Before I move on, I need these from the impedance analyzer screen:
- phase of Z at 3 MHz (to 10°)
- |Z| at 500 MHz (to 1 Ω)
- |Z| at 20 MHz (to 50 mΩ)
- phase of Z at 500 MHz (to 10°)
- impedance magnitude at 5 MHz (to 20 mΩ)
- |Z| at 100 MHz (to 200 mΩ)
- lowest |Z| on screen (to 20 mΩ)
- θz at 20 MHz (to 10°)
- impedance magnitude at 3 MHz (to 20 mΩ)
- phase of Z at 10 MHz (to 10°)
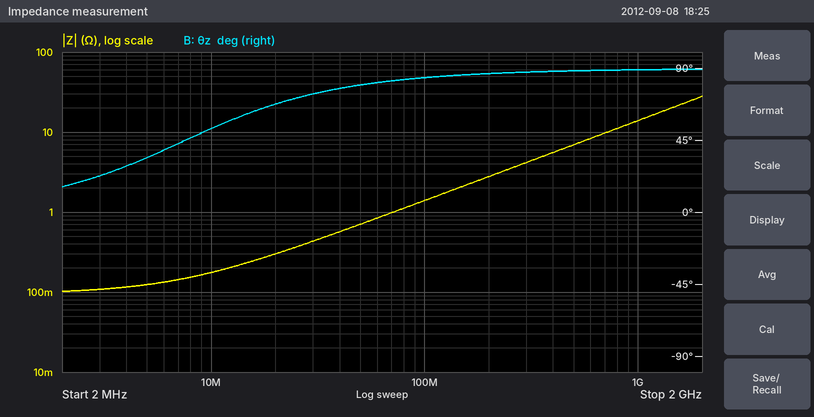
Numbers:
20°
7 Ω
300 mΩ
90°
120 mΩ
1.4 Ω
100 mΩ
70°
100 mΩ
50°
